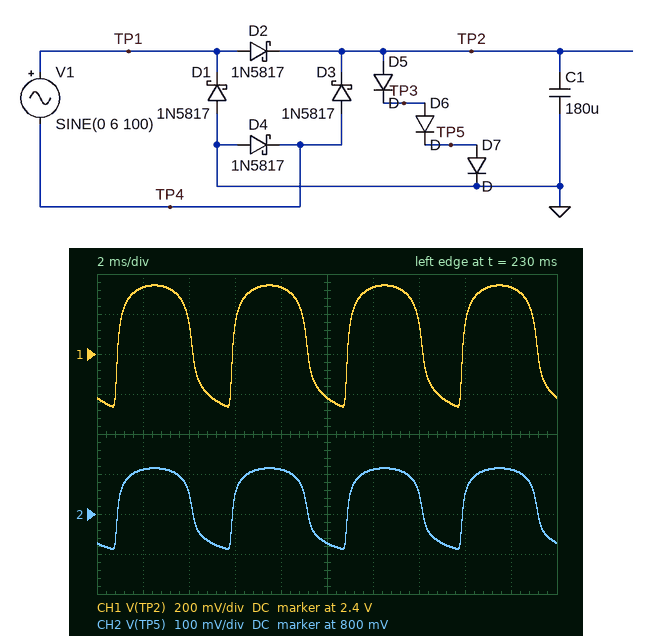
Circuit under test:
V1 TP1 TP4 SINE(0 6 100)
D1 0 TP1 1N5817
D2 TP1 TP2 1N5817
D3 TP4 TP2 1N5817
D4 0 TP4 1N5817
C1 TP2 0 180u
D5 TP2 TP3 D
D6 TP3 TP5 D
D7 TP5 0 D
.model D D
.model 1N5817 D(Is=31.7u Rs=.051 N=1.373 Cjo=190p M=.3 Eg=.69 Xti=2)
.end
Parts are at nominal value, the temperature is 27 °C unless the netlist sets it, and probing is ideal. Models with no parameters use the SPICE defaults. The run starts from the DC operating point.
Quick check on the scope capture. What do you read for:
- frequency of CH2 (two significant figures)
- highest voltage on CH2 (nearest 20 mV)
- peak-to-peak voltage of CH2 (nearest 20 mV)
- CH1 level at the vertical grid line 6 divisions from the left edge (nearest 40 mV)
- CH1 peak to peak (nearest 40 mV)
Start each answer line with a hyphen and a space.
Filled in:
- 200 Hz
- 920 mV
- 200 mV
- 2.72 V
- 600 mV
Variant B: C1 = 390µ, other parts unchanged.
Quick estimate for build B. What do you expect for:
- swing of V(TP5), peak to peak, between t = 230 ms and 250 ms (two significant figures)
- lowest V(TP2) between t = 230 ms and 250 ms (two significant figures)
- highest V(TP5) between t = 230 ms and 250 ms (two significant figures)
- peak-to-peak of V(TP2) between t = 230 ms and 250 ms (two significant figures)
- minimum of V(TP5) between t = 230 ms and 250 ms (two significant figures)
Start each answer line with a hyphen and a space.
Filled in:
- 180 mV
- 2.2 V
- 910 mV
- 550 mV
- 730 mV
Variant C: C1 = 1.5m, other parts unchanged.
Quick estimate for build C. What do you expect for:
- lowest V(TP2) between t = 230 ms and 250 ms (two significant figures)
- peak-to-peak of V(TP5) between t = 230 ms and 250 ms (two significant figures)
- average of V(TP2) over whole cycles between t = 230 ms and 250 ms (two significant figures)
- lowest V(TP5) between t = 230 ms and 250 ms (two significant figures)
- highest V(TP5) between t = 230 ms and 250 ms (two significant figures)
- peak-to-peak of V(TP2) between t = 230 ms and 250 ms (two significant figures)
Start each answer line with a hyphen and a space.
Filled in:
- 2.3 V
- 150 mV
- 2.6 V
- 760 mV
- 910 mV
- 450 mV
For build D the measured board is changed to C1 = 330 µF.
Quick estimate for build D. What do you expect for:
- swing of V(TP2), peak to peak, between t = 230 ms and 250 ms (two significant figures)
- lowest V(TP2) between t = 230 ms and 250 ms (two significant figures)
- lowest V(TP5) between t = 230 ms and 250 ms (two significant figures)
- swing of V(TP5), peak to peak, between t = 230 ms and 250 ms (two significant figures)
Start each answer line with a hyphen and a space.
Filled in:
- 560 mV
- 2.2 V
- 730 mV
- 190 mV
